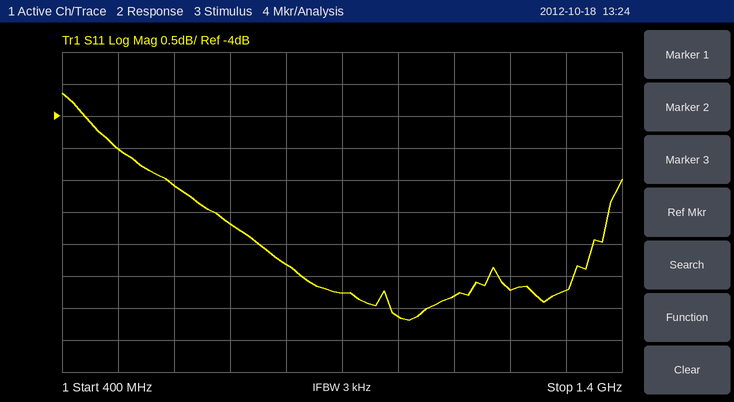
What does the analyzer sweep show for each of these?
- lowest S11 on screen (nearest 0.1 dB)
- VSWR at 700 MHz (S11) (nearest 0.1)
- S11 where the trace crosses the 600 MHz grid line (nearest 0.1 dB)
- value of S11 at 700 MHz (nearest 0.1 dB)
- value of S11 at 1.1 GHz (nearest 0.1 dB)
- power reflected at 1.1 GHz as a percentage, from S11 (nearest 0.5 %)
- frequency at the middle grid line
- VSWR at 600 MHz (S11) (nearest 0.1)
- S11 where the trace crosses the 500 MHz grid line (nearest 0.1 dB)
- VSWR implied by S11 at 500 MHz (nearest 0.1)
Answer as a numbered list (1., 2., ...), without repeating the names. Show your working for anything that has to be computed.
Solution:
1. -7.2 dB
2. |Γ| = 10^(-5.7/20) = 0.5188; VSWR = (1 + 0.5188)/(1 − 0.5188) ≈ 3.2
3. -5.1 dB
4. -5.7 dB
5. -6.8 dB
6. 10^(-6.8/10) ≈ 20.9 %, so 21.0 % to the nearest 0.5 %
7. 900 MHz
8. |Γ| = 10^(-5.1/20) = 0.5559; VSWR = (1 + 0.5559)/(1 − 0.5559) ≈ 3.5
9. -4.5 dB
10. |Γ| = 10^(-4.5/20) = 0.5957; VSWR = (1 + 0.5957)/(1 − 0.5957) ≈ 3.9
